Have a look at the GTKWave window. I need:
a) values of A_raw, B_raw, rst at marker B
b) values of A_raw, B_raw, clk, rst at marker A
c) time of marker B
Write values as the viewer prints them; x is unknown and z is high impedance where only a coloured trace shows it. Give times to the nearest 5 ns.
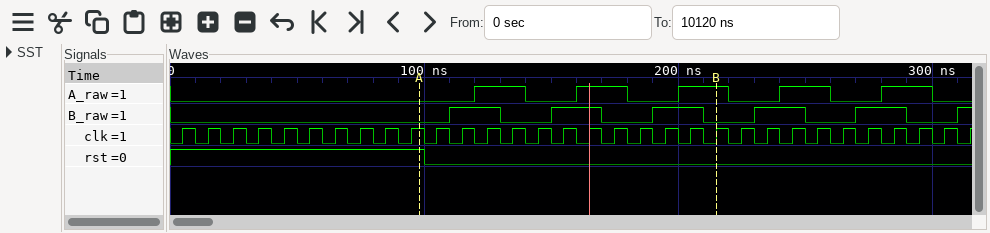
A_raw=1, B_raw=0, rst=0
A_raw=0, B_raw=0, clk=1, rst=1
215 ns
